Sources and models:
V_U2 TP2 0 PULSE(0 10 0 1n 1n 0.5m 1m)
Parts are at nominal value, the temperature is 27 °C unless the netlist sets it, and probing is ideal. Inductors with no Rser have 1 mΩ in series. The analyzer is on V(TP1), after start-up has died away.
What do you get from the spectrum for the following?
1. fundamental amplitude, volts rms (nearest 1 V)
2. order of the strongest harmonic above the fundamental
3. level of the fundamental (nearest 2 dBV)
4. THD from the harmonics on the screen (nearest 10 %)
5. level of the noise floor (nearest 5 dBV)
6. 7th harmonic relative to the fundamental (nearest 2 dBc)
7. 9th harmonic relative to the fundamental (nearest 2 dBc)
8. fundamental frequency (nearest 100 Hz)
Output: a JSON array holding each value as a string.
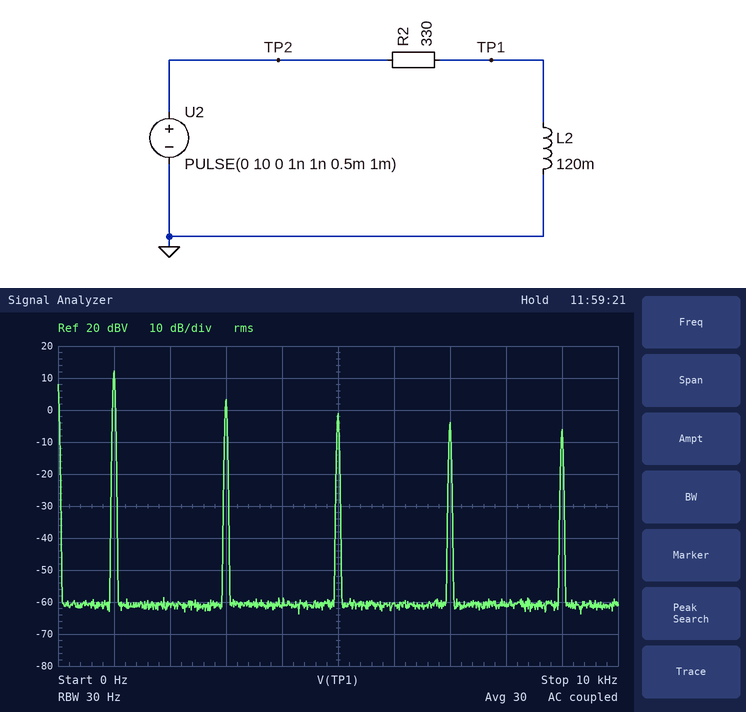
["4 V", "3", "12 dBV", "50 %", "-60 dBV", "-16 dBc", "-18 dBc", "1.0 kHz"]
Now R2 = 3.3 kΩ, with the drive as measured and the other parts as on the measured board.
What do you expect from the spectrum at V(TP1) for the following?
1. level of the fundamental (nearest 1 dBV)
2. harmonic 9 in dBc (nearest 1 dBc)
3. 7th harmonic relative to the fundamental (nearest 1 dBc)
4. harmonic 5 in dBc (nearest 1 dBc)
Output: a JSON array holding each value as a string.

["0 dBV", "-7 dBc", "-5 dBc", "-3 dBc"]
